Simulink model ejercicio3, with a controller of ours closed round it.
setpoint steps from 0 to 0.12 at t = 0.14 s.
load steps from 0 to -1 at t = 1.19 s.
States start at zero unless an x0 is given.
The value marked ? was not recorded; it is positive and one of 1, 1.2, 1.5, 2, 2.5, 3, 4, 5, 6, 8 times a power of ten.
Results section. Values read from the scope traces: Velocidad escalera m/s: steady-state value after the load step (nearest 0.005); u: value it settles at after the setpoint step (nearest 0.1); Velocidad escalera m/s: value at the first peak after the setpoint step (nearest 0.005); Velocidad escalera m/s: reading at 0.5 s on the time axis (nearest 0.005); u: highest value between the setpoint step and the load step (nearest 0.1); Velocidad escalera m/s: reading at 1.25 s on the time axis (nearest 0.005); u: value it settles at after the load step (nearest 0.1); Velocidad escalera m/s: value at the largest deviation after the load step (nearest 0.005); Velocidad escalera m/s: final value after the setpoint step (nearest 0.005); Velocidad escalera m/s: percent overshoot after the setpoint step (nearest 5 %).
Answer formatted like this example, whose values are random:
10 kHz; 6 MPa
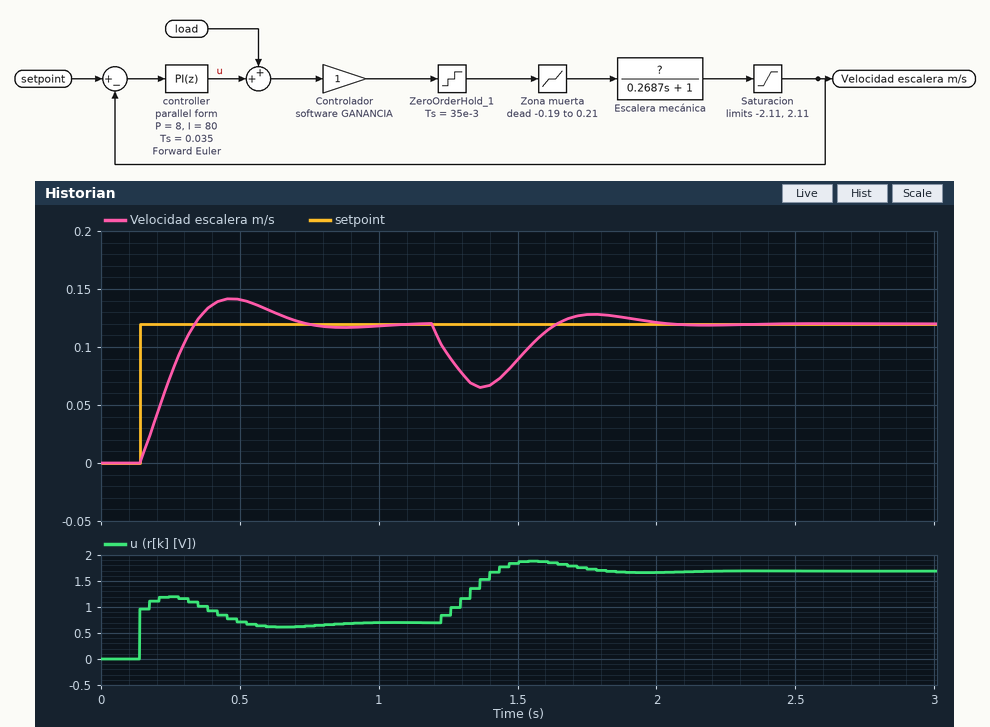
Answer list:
0.120; 0.7; 0.140; 0.140; 1.2; 0.095; 1.7; 0.065; 0.120; 20 %
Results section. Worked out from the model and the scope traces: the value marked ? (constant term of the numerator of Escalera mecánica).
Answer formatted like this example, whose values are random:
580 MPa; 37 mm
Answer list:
0.25
